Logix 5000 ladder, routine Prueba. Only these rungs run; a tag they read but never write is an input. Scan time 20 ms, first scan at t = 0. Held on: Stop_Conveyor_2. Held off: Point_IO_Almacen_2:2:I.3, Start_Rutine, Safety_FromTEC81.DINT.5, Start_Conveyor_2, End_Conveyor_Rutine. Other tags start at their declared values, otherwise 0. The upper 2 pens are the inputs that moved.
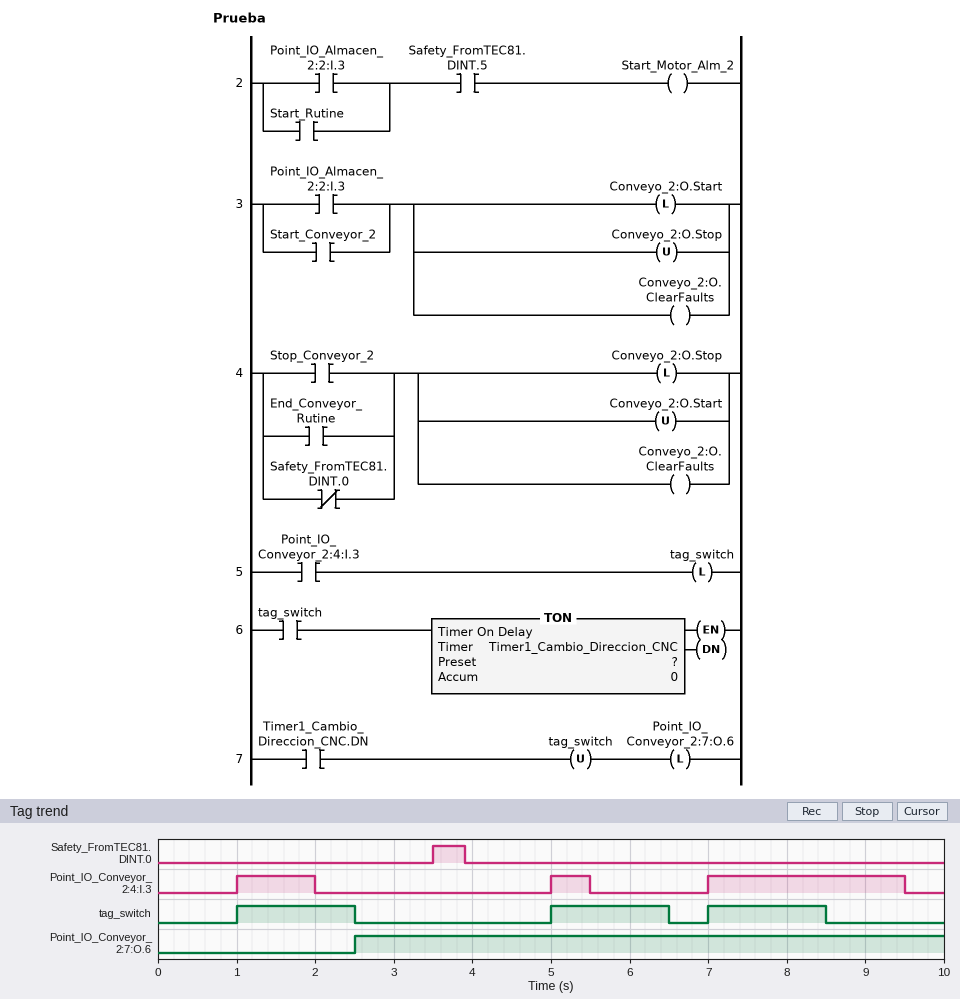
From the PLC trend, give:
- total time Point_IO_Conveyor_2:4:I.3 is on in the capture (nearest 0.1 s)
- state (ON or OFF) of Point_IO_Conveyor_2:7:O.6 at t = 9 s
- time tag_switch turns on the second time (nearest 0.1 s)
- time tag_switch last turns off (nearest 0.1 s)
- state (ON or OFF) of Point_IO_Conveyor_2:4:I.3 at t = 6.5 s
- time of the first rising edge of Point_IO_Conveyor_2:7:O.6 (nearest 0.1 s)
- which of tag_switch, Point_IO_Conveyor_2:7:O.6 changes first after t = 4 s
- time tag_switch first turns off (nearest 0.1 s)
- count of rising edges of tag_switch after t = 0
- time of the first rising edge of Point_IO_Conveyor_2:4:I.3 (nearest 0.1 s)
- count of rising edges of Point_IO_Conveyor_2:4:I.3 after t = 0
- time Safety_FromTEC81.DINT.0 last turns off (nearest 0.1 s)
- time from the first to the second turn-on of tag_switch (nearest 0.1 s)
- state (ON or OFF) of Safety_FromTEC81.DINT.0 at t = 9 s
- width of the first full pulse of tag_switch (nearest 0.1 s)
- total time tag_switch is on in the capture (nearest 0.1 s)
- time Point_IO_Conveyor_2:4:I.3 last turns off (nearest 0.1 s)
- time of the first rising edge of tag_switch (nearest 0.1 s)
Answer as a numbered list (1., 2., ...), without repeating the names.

1. 4.0 s
2. ON
3. 5.0 s
4. 8.5 s
5. OFF
6. 2.5 s
7. tag_switch
8. 2.5 s
9. 3
10. 1.0 s
11. 3
12. 3.9 s
13. 4.0 s
14. OFF
15. 1.5 s
16. 4.5 s
17. 9.5 s
18. 1.0 s
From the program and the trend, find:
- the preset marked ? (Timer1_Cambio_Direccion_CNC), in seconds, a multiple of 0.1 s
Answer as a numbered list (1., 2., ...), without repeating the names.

1. 1.5 s
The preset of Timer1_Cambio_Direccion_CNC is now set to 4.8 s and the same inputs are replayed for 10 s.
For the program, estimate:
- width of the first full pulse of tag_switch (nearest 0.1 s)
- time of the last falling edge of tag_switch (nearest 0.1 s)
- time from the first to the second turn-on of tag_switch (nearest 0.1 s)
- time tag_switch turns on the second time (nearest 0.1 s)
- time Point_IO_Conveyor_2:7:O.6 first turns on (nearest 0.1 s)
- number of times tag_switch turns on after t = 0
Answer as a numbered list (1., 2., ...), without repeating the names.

1. 4.8 s
2. 5.8 s
3. 6.0 s
4. 7.0 s
5. 5.8 s
6. 2
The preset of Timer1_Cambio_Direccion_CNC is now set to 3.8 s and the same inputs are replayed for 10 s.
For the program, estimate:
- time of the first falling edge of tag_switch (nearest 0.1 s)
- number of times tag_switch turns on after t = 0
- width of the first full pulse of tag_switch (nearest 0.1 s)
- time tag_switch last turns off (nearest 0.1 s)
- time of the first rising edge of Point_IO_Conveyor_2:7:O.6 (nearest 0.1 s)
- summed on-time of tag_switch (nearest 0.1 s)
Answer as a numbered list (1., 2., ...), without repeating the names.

1. 4.8 s
2. 2
3. 3.8 s
4. 8.8 s
5. 4.8 s
6. 7.6 s
